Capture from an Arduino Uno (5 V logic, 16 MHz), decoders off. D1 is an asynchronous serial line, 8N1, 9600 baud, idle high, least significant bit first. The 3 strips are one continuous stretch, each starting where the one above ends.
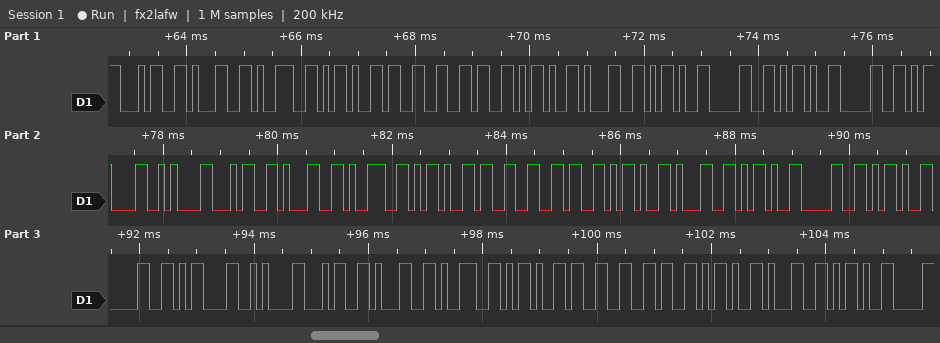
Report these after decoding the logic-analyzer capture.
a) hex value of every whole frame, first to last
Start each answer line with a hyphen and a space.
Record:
- 34 31 39 2D 33 36 2D 31 2D 30 2D 30 0D 0A 34 31 39 2D 33 36 2D 31 2D 30 2D 30 0D 0A 34 31 39 2D 33 36 2D 31 2D
